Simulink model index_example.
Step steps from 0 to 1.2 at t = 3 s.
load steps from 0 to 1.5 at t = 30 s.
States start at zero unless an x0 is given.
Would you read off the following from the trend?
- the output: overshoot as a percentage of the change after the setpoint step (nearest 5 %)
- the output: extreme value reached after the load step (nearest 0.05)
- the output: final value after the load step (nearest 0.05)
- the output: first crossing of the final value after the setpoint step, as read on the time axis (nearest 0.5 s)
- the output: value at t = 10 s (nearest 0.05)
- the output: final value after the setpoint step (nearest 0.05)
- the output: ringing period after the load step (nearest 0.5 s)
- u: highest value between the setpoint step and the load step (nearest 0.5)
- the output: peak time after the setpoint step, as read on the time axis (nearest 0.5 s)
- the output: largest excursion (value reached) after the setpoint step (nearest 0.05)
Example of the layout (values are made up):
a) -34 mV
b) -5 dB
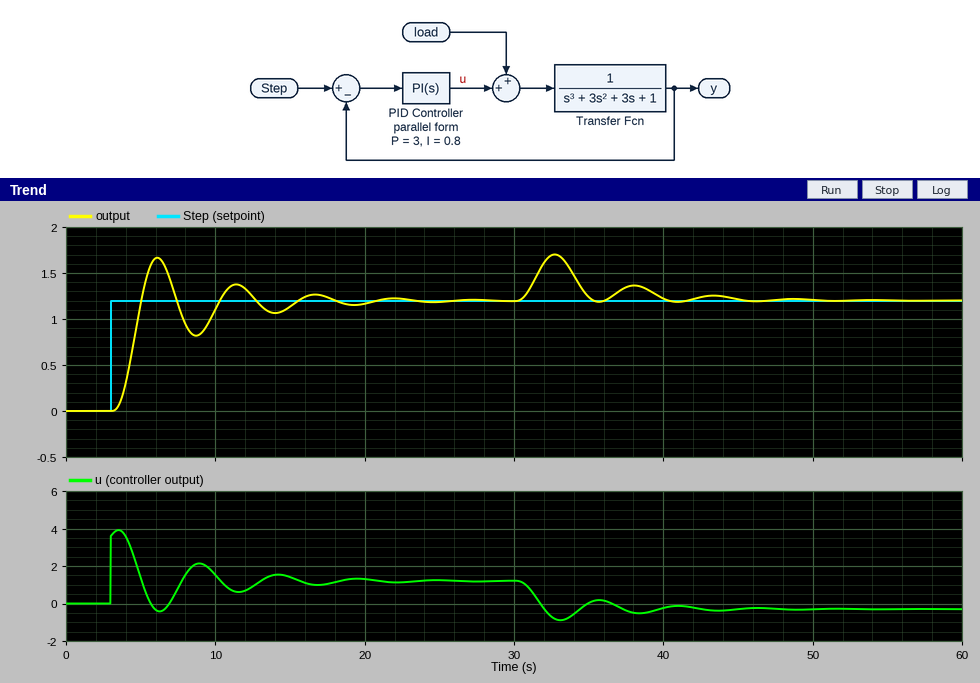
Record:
a) 40 %
b) 1.70
c) 1.20
d) 5.0 s
e) 1.10
f) 1.20
g) 5.5 s
h) 4.0
i) 6.0 s
j) 1.65
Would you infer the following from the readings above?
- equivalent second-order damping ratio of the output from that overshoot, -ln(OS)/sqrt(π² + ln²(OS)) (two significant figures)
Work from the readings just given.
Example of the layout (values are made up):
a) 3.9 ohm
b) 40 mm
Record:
a) 0.28
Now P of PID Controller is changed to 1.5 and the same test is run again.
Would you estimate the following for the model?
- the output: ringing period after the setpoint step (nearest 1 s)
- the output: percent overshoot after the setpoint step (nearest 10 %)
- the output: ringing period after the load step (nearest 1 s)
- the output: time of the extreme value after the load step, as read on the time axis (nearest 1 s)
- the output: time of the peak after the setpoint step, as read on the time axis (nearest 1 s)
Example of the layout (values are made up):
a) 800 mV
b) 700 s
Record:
a) 7 s
b) 30 %
c) 8 s
d) 33 s
e) 7 s
